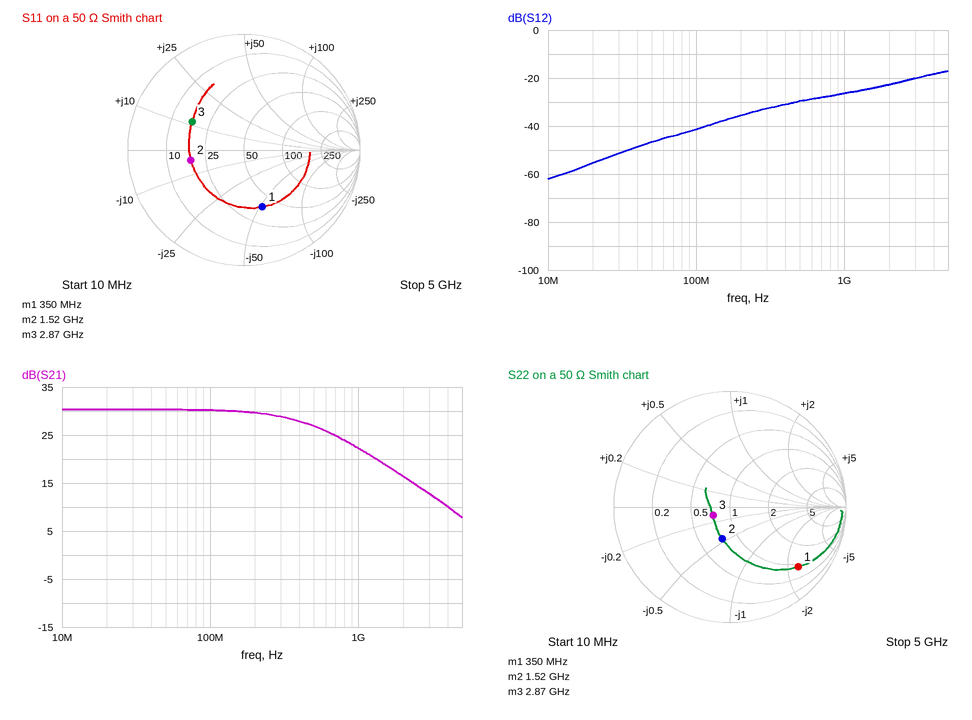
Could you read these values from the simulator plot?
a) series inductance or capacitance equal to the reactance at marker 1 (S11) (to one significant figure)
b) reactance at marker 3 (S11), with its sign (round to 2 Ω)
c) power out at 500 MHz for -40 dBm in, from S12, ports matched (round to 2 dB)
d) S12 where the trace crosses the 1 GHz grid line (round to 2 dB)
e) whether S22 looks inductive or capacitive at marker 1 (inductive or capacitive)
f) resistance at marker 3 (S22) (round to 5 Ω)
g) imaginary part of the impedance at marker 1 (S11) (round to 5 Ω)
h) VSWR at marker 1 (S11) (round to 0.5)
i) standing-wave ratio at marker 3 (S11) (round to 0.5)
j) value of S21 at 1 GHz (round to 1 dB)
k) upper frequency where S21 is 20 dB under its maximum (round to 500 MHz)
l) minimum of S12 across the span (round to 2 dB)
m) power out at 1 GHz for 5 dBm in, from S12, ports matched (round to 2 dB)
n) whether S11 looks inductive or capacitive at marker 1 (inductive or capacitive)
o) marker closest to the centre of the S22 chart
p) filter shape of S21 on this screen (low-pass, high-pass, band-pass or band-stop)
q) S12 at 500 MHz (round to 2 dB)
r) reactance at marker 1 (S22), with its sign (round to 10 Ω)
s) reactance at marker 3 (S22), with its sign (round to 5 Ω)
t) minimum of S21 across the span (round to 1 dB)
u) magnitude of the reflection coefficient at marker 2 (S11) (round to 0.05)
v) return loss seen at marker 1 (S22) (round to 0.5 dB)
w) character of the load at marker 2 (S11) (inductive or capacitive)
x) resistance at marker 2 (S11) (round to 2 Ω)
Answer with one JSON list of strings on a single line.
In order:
["9 pF", "+12 Ω", "-70 dBm", "-26 dB", "capacitive", "35 Ω", "-50 Ω", "3.0", "3.0", "22 dB", "4.0 GHz", "-62 dB", "-22 dBm", "capacitive", "marker 3", "low-pass", "-30 dB", "-120 Ω", "-5 Ω", "8 dB", "0.45", "2.0 dB", "capacitive", "18 Ω"]
